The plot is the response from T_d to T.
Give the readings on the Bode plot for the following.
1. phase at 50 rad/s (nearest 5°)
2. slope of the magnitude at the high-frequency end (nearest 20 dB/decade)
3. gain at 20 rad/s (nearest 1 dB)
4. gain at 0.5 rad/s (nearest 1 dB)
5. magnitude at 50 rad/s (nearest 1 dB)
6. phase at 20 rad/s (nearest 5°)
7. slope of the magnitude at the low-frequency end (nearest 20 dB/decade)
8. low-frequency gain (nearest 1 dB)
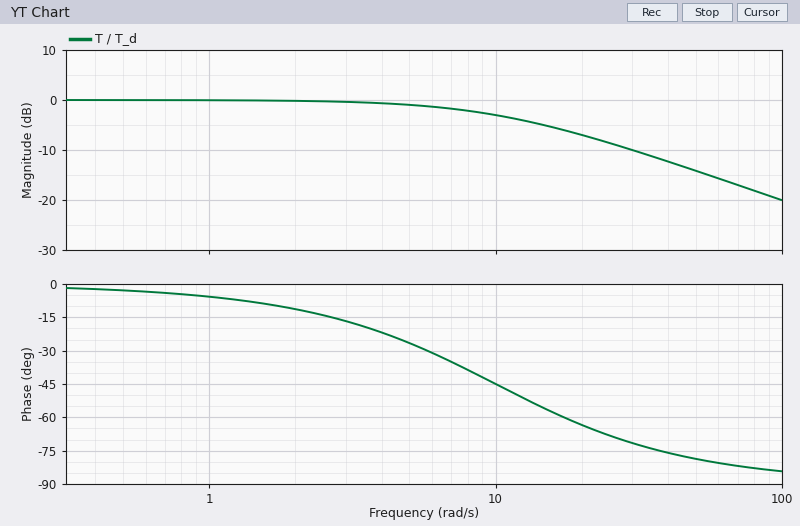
-80°
-20 dB/decade
-7 dB
0 dB
-14 dB
-65°
0 dB/decade
0 dB
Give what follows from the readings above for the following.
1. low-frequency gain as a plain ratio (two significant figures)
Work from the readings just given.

1.0
